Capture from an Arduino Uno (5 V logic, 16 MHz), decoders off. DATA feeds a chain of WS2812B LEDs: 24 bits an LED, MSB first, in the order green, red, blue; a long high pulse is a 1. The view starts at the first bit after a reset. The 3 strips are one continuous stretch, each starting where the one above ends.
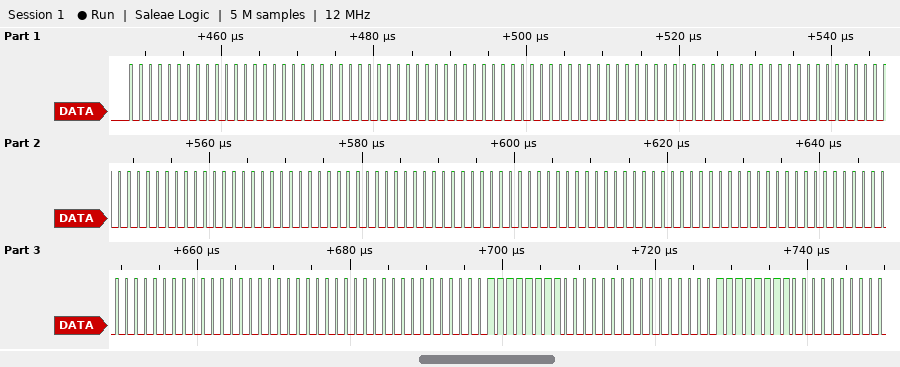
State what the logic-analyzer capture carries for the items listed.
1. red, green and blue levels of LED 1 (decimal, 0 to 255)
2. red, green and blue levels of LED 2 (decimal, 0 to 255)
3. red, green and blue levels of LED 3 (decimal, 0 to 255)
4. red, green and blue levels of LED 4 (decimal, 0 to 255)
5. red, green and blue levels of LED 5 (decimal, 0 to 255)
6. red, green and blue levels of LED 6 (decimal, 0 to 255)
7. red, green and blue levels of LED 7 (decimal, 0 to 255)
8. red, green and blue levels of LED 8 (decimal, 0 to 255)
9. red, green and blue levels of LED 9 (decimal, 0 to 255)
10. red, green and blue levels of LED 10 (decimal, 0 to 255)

0, 0, 0
0, 0, 0
0, 0, 0
0, 0, 0
0, 0, 0
0, 0, 0
0, 0, 0
0, 0, 0
255, 0, 0
255, 0, 0
